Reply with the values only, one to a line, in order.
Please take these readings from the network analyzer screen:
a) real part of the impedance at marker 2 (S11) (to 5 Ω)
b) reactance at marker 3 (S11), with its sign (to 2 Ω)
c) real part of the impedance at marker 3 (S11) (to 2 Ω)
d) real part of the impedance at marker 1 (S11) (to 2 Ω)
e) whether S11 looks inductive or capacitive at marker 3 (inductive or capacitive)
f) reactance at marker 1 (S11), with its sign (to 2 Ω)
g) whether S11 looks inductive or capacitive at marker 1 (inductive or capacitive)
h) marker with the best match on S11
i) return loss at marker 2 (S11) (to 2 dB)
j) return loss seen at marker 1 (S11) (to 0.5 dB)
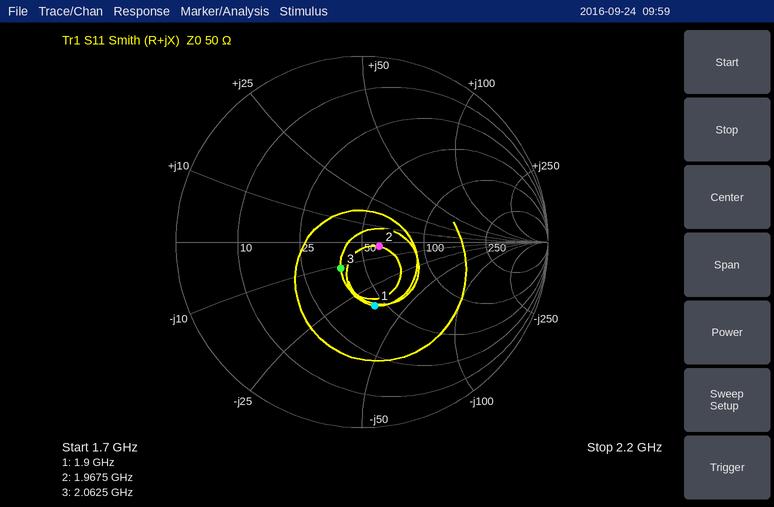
60 Ω
-12 Ω
38 Ω
44 Ω
capacitive
-34 Ω
capacitive
marker 2
20 dB
9.0 dB
